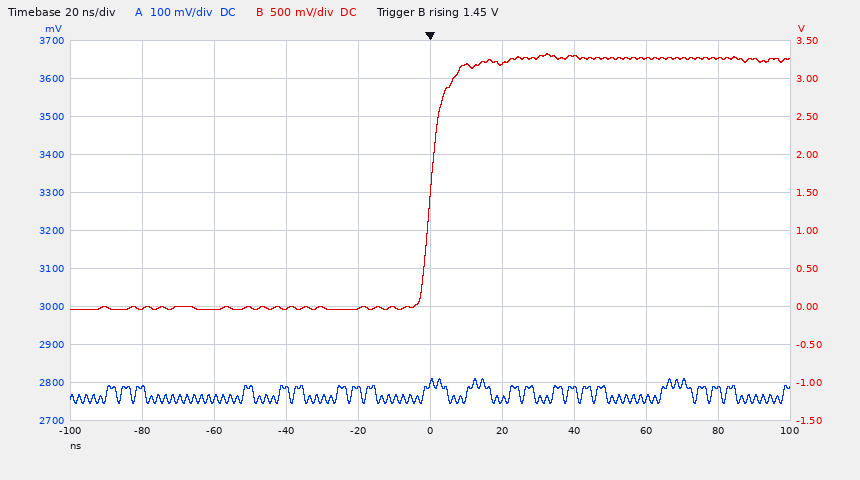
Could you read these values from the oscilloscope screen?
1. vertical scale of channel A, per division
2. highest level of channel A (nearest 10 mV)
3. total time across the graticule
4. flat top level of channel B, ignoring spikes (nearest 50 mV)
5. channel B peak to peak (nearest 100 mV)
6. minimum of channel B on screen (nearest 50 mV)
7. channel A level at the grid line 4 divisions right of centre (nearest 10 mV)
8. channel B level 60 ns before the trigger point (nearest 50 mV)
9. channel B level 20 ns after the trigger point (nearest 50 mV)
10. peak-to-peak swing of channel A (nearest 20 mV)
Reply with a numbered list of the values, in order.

1. 100 mV
2. 2.81 V
3. 200 ns
4. 3.25 V
5. 3.40 V
6. -50 mV
7. 2.78 V
8. -50 mV
9. 3.20 V
10. 60 mV
